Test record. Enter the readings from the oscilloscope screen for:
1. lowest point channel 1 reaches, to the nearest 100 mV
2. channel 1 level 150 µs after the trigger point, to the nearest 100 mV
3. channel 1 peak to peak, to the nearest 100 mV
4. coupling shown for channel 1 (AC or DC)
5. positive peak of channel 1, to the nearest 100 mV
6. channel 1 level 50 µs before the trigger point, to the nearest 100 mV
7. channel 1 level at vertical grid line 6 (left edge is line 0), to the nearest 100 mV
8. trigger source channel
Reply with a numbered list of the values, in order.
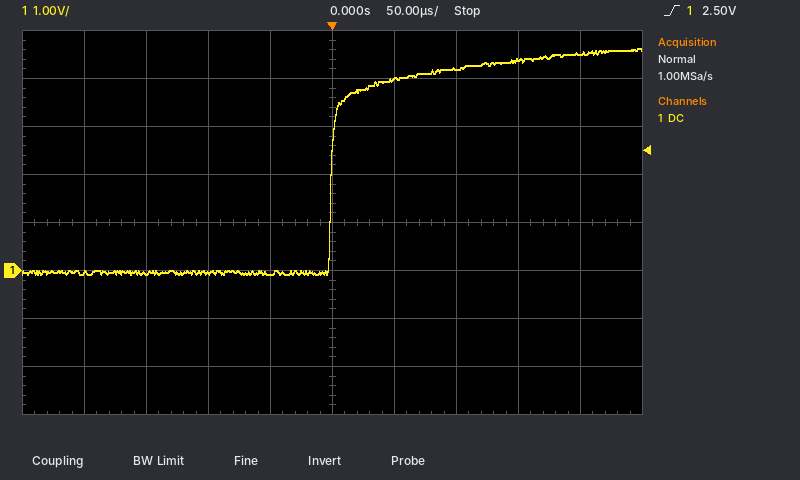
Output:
1. -100 mV
2. 4.4 V
3. 4.7 V
4. DC
5. 4.6 V
6. -100 mV
7. 4.0 V
8. channel 1
